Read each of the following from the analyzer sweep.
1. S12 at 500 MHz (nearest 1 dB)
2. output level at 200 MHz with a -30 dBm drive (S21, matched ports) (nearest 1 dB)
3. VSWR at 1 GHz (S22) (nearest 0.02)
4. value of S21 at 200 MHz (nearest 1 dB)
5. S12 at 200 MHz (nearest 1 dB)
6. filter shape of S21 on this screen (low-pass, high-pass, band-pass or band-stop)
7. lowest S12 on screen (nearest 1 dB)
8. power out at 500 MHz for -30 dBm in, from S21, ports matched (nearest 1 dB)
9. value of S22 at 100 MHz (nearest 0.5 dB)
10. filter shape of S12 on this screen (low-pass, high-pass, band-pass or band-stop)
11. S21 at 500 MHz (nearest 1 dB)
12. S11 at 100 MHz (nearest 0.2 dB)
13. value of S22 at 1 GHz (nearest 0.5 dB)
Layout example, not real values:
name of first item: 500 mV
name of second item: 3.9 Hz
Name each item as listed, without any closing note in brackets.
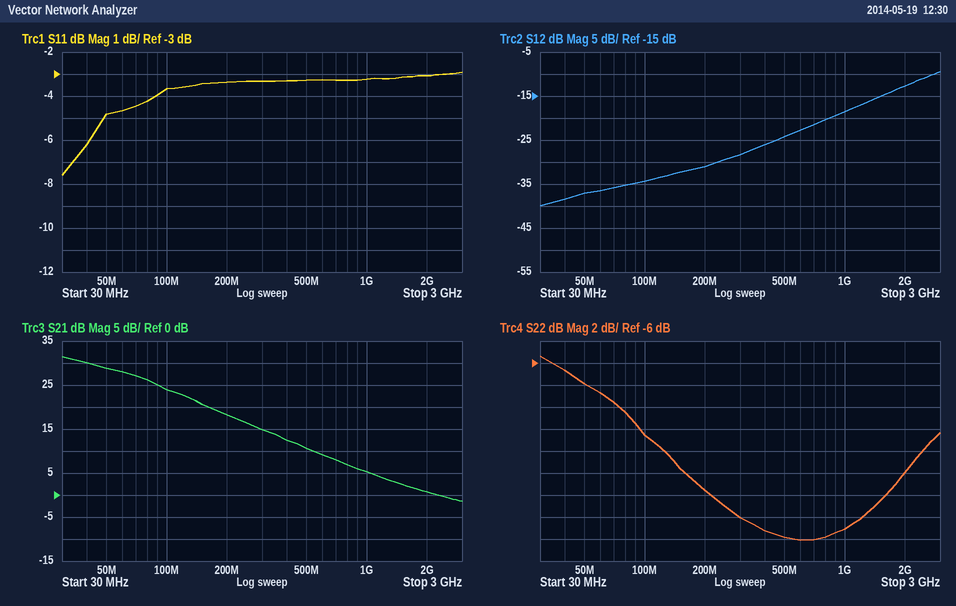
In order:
S12 at 500 MHz: -24 dB
output level at 200 MHz with a -30 dBm drive (S21, matched ports): -12 dBm
VSWR at 1 GHz (S22): 1.20
value of S21 at 200 MHz: 18 dB
S12 at 200 MHz: -31 dB
filter shape of S21 on this screen: low-pass
lowest S12 on screen: -40 dB
power out at 500 MHz for -30 dBm in, from S21, ports matched: -19 dBm
value of S22 at 100 MHz: -12.5 dB
filter shape of S12 on this screen: high-pass
S21 at 500 MHz: 11 dB
S11 at 100 MHz: -3.6 dB
value of S22 at 1 GHz: -21.0 dB
